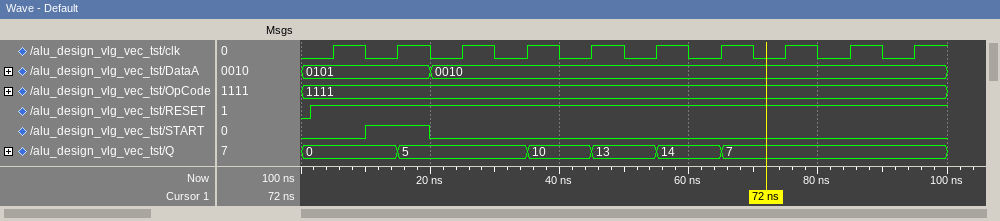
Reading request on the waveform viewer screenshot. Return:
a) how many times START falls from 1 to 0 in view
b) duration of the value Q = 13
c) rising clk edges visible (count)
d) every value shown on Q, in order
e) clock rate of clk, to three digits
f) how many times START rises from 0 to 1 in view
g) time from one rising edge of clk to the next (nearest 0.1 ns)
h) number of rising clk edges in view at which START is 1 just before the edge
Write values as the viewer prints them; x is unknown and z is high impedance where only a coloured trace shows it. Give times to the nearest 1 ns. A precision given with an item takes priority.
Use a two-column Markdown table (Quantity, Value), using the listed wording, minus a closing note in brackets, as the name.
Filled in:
| Quantity | Value |
|---|---|
| how many times START falls from 1 to 0 in view | 1 |
| duration of the value Q = 13 | 10 ns |
| rising clk edges visible | 10 |
| every value shown on Q, in order | 0, 5, 10, 13, 14, 7 |
| clock rate of clk, to three digits | 100 MHz |
| how many times START rises from 0 to 1 in view | 1 |
| time from one rising edge of clk to the next | 10 ns |
| number of rising clk edges in view at which START is 1 just before the edge | 1 |
